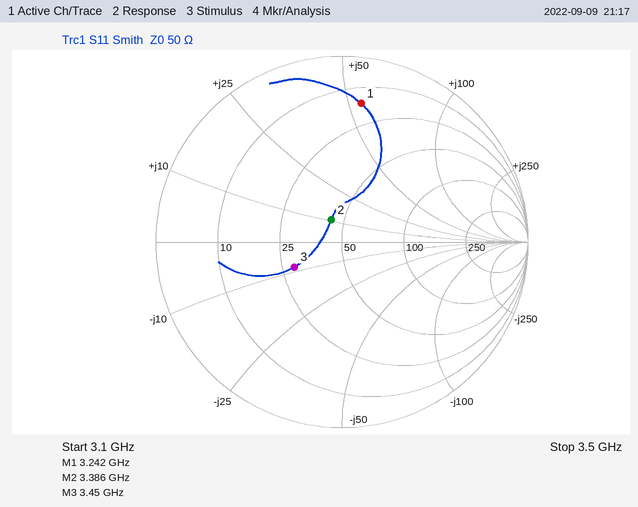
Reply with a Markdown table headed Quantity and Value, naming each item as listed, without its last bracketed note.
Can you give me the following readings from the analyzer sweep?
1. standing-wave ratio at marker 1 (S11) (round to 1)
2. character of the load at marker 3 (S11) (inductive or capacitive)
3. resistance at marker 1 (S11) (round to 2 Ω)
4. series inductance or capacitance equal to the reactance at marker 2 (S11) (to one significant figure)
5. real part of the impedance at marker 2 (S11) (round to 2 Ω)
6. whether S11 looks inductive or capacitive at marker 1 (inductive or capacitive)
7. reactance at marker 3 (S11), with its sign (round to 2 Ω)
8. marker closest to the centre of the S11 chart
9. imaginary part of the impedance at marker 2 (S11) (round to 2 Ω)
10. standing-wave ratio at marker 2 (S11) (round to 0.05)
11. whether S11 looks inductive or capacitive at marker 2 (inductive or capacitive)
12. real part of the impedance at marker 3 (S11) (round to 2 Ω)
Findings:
| Quantity | Value |
|---|---|
| standing-wave ratio at marker 1 (S11) | 7 |
| character of the load at marker 3 (S11) | capacitive |
| resistance at marker 1 (S11) | 16 Ω |
| series inductance or capacitance equal to the reactance at marker 2 (S11) | 500 pH |
| real part of the impedance at marker 2 (S11) | 44 Ω |
| whether S11 looks inductive or capacitive at marker 1 | inductive |
| reactance at marker 3 (S11), with its sign | -8 Ω |
| marker closest to the centre of the S11 chart | marker 2 |
| imaginary part of the impedance at marker 2 (S11) | +10 Ω |
| standing-wave ratio at marker 2 (S11) | 1.30 |
| whether S11 looks inductive or capacitive at marker 2 | inductive |
| real part of the impedance at marker 3 (S11) | 28 Ω |
